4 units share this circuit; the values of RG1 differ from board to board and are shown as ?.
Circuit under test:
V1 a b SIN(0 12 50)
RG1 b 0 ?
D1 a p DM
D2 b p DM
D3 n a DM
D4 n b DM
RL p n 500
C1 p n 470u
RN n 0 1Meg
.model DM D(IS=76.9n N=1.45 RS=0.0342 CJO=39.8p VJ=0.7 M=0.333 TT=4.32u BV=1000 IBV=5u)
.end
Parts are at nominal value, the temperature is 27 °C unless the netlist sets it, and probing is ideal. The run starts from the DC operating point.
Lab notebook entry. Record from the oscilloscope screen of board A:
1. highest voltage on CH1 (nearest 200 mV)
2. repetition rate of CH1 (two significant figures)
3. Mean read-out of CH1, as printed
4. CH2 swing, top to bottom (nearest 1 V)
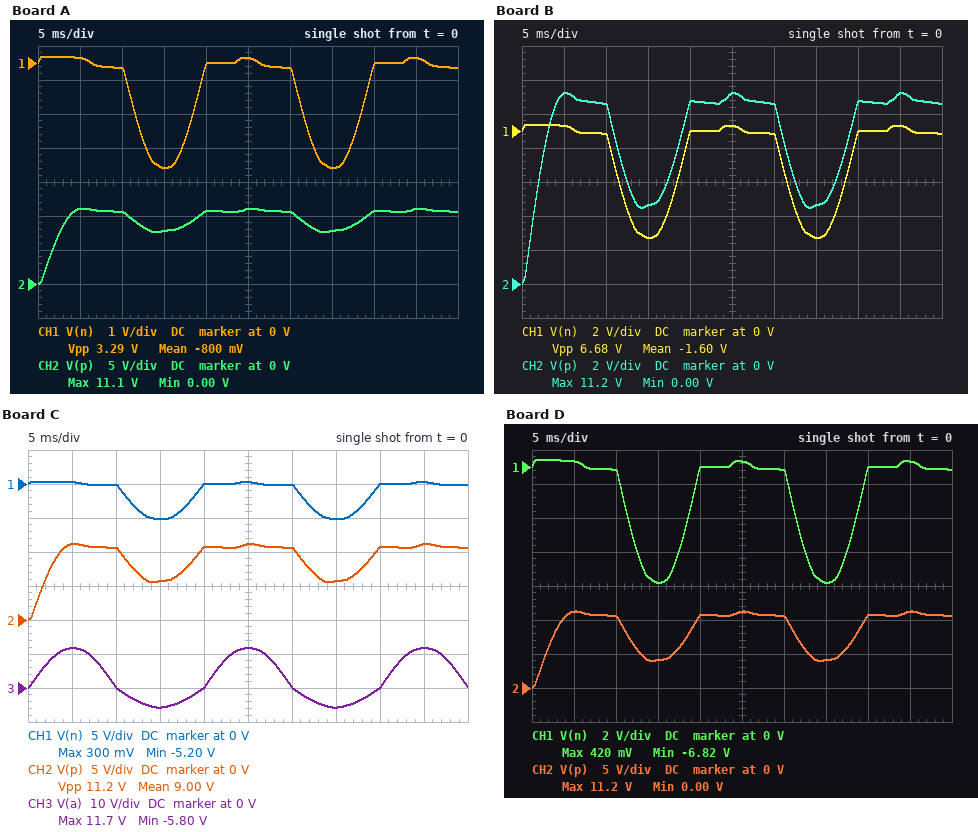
200 mV
50 Hz
-800 mV
11 V
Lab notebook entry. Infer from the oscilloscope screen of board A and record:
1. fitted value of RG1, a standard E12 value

2.7 MΩ
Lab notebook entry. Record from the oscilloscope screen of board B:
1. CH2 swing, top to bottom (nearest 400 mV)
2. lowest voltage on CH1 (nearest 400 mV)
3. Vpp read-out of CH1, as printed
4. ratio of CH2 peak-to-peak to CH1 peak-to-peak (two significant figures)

11.2 V
-6.4 V
6.68 V
1.7
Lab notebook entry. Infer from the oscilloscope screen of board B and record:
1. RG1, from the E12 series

820 kΩ
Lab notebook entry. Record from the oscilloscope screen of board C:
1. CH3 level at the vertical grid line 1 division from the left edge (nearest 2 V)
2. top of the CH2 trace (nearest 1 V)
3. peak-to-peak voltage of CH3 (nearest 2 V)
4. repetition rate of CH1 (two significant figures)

12 V
11 V
18 V
50 Hz
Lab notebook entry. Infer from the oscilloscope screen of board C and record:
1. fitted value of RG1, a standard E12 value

1.2 MΩ
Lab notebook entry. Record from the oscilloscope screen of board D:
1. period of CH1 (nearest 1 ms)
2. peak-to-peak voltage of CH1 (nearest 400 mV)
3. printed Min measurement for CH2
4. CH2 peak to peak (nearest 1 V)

20 ms
7.2 V
0.00 V
11 V
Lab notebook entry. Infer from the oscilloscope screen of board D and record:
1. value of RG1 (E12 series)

680 kΩ
